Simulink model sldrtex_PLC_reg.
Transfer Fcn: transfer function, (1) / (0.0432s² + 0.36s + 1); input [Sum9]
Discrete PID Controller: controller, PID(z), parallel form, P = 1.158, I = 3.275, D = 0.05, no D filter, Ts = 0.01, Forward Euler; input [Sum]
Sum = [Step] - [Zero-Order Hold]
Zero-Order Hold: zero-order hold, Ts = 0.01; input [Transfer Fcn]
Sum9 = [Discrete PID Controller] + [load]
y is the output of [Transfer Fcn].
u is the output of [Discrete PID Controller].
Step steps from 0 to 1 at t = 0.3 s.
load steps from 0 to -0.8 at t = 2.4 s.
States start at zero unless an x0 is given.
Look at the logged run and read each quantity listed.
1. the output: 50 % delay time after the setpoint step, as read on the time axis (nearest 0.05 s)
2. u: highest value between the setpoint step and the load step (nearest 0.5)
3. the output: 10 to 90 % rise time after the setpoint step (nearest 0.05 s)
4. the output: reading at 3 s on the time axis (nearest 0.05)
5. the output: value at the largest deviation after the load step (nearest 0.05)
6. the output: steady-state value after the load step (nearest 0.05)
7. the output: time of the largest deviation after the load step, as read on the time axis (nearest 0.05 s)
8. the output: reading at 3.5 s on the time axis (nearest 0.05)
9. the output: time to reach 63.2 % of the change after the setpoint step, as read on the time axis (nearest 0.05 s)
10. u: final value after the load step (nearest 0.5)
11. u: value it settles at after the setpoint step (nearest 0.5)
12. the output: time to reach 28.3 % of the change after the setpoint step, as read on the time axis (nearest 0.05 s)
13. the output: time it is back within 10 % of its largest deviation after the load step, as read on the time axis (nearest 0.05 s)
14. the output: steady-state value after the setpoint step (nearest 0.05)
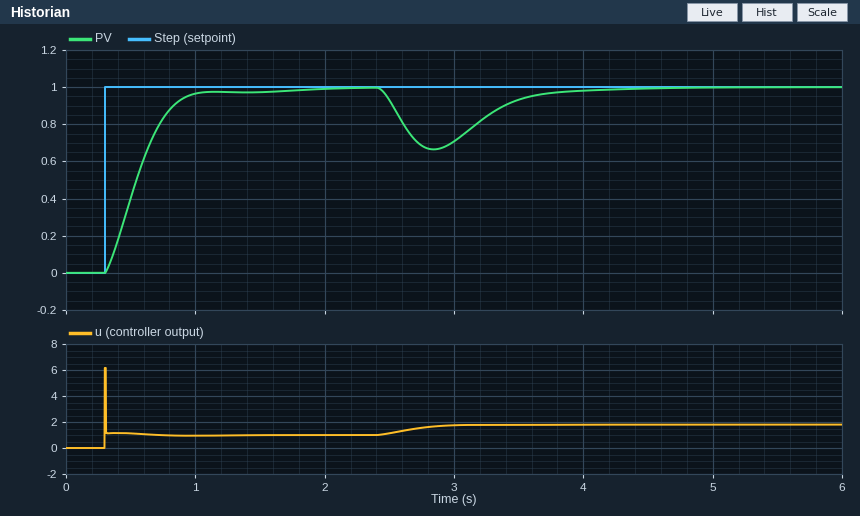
0.55 s
6.0
0.45 s
0.70
0.65
1.00
2.85 s
0.95
0.60 s
2.0
1.0
0.45 s
3.75 s
1.00
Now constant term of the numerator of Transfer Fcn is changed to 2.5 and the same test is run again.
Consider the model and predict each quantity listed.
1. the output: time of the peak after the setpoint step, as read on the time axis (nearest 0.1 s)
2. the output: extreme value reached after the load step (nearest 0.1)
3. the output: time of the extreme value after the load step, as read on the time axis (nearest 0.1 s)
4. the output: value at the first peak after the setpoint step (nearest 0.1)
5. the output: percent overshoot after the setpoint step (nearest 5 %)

0.7 s
0.5
2.7 s
1.1
10 %
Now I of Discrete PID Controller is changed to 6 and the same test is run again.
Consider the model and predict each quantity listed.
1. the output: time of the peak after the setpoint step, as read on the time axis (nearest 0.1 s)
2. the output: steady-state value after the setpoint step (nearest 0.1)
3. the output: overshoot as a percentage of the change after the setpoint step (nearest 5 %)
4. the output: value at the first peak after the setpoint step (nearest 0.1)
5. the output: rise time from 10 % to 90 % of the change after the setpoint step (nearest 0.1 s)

1.0 s
1.0
20 %
1.2
0.3 s
